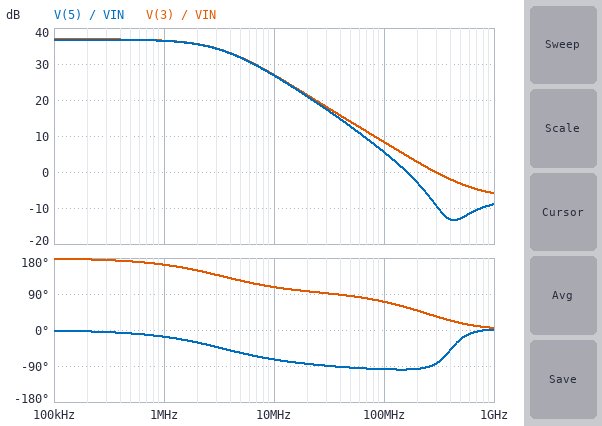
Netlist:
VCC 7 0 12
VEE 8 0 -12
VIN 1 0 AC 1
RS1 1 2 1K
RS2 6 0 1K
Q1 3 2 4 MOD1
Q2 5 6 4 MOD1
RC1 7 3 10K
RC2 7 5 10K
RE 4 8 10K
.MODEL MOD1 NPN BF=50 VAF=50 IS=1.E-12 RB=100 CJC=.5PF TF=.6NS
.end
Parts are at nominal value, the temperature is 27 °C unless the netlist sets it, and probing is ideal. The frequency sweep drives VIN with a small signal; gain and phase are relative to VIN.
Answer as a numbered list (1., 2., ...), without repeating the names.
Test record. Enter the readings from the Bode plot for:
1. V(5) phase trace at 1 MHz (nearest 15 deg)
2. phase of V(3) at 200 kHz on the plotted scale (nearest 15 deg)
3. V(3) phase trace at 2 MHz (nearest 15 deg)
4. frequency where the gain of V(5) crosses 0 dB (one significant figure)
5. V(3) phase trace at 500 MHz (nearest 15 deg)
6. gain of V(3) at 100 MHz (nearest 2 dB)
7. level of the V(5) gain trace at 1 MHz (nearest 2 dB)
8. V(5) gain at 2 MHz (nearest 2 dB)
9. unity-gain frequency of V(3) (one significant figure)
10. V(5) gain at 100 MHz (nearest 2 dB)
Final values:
1. -15 deg
2. 180 deg
3. 150 deg
4. 200 MHz
5. 15 deg
6. 8 dB
7. 36 dB
8. 36 dB
9. 300 MHz
10. 6 dB
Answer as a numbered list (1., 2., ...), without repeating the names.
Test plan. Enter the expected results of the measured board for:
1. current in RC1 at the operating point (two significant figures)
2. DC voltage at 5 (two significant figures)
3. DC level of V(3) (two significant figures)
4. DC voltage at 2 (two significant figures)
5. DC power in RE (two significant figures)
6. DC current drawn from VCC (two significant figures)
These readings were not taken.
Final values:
1. 560 µA
2. 6.4 V
3. 6.4 V
4. -10 mV
5. 13 mW
6. 1.1 mA
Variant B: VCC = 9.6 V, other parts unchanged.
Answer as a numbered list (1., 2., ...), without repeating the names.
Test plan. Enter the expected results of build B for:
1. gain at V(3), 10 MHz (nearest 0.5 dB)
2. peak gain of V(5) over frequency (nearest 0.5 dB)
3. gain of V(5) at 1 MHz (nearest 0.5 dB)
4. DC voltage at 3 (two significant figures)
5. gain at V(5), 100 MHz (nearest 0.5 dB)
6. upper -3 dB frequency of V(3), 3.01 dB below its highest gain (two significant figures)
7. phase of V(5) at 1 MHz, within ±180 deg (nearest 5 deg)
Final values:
1. 26.0 dB
2. 36.5 dB
3. 36.0 dB
4. 4.0 V
5. 4.5 dB
6. 3.1 MHz
7. -20 deg
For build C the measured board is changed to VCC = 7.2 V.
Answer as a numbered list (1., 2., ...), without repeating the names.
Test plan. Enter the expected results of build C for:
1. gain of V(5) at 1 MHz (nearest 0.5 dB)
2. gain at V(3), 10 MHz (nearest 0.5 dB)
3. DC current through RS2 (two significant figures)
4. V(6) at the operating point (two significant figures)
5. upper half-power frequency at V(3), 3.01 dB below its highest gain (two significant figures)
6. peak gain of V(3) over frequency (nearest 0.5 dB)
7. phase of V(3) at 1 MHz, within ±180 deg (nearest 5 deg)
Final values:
1. 36.0 dB
2. 24.5 dB
3. 11 µA
4. -11 mV
5. 2.6 MHz
6. 36.5 dB
7. 160 deg
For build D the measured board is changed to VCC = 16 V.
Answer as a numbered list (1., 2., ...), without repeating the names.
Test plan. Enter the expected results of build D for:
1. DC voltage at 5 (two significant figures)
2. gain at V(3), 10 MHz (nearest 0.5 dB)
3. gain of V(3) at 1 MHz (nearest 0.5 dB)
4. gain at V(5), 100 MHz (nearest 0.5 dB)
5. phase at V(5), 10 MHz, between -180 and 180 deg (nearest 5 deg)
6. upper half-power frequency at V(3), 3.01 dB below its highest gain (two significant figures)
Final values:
1. 10 V
2. 28.0 dB
3. 37.0 dB
4. 6.5 dB
5. -70 deg
6. 3.7 MHz
